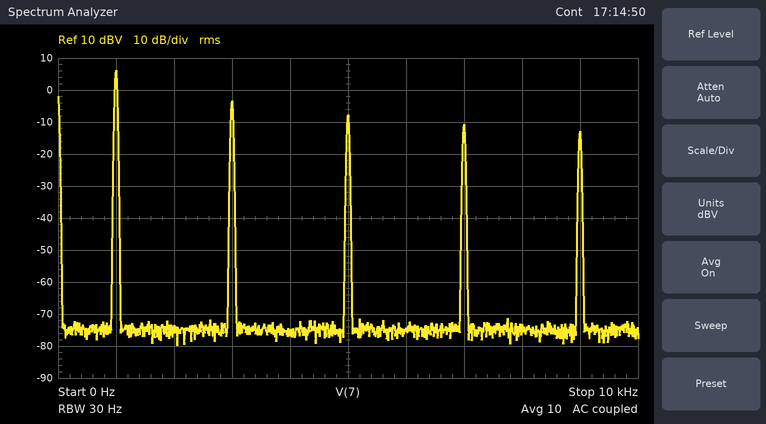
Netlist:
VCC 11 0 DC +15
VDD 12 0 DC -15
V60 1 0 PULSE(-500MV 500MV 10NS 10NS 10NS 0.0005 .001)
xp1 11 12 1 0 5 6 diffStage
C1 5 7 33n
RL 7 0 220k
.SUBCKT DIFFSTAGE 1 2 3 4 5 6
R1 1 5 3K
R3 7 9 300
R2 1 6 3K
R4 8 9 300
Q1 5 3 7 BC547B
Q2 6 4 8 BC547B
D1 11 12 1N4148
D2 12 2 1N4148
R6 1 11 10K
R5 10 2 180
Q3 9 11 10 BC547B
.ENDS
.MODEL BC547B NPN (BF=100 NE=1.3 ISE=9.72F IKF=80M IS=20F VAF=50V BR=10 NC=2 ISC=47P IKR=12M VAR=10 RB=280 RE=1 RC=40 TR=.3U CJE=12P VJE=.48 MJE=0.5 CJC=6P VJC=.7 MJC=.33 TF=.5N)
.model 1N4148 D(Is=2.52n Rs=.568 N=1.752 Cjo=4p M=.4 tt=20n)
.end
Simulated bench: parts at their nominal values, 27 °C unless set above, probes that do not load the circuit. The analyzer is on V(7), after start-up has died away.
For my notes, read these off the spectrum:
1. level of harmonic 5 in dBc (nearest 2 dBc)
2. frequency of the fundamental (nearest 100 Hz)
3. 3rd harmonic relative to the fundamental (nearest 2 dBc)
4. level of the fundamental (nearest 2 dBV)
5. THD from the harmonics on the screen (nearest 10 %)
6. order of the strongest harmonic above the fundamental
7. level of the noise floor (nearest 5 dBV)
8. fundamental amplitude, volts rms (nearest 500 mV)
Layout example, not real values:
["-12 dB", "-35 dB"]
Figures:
["-14 dBc", "1.0 kHz", "-10 dBc", "6 dBV", "40 %", "3", "-75 dBV", "2.0 V"]
